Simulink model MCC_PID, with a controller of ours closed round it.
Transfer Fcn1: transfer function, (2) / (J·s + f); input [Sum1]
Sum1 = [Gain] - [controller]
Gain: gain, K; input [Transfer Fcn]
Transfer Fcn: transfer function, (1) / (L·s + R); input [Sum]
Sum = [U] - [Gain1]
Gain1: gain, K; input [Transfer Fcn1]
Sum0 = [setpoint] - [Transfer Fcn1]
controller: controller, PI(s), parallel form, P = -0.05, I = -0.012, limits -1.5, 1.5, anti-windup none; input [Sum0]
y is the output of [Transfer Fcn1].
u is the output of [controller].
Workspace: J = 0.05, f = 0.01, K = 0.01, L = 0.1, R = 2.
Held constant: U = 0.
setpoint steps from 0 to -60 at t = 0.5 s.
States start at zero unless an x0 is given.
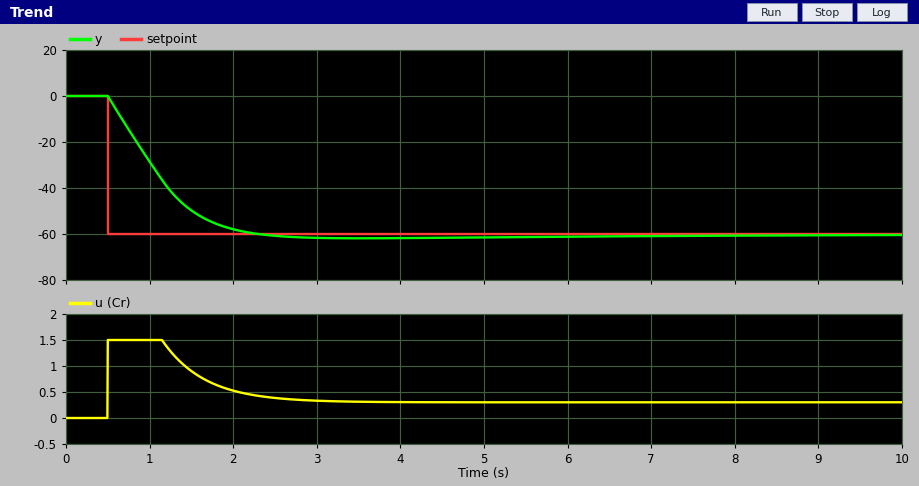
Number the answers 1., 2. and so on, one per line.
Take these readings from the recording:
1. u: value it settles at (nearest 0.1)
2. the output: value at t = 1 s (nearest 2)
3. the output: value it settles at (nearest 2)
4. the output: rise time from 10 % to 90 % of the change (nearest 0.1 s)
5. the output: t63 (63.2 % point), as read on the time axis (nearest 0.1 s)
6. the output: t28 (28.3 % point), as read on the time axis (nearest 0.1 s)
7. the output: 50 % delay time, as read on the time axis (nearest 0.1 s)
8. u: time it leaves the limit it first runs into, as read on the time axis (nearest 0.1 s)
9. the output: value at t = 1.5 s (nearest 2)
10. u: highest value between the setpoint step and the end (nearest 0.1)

1. 0.3
2. -28
3. -60
4. 1.1 s
5. 1.2 s
6. 0.8 s
7. 1.0 s
8. 1.2 s
9. -50
10. 1.5
